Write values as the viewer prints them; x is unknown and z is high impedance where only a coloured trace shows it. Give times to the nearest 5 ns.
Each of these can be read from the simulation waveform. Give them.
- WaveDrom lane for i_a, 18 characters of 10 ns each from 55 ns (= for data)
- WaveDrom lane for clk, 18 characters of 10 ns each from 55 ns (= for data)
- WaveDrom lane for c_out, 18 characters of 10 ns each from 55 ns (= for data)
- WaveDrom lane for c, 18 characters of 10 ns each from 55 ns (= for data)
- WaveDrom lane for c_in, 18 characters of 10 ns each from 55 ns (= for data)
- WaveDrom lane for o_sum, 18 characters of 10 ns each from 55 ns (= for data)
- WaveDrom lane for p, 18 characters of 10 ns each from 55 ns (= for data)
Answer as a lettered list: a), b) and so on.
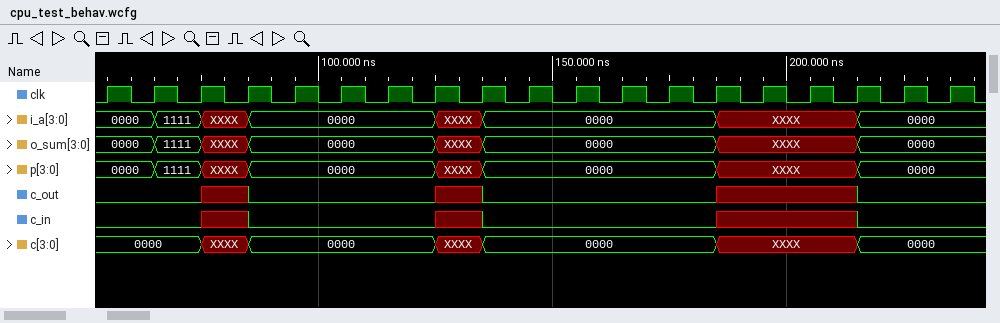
a) {name: 'i_a', wave: '==x=...x=....x..=.', data: '0000 1111 0000 0000 0000'}
b) {name: 'clk', wave: 'p.................'}
c) {name: 'c_out', wave: '0.x0...x0....x..0.'}
d) {name: 'c', wave: '=.x=...x=....x..=.', data: '0000 0000 0000 0000'}
e) {name: 'c_in', wave: '0.x0...x0....x..0.'}
f) {name: 'o_sum', wave: '==x=...x=....x..=.', data: '0000 1111 0000 0000 0000'}
g) {name: 'p', wave: '==x=...x=....x..=.', data: '0000 1111 0000 0000 0000'}
